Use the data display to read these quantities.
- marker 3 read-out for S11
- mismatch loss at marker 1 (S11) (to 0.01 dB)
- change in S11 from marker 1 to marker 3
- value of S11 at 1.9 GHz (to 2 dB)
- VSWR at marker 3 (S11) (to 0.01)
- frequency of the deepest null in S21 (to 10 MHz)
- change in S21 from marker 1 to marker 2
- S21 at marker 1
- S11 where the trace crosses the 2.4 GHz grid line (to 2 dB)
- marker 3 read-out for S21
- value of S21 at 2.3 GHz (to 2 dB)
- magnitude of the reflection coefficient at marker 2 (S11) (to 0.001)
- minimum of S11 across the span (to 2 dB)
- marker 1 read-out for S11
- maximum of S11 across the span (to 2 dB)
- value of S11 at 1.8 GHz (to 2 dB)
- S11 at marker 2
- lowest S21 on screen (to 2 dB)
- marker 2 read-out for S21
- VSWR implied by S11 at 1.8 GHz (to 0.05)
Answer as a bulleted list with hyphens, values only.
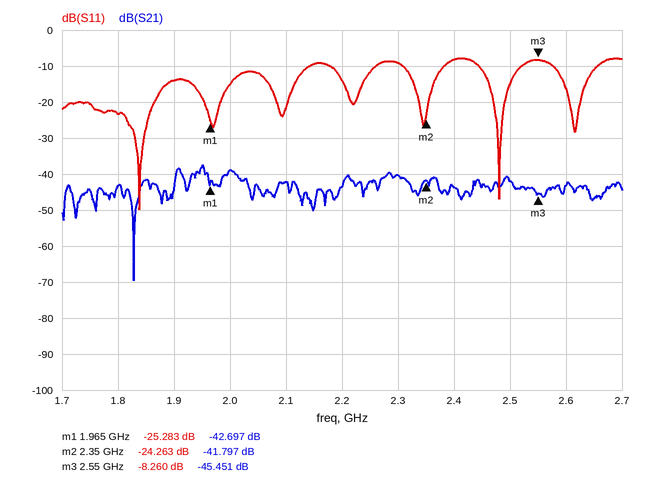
- -8.260 dB
- 0.01 dB
- 17.023 dB
- -14 dB
- 2.26
- 1.83 GHz
- 0.900 dB
- -42.697 dB
- -8 dB
- -45.451 dB
- -40 dB
- 0.061
- -50 dB
- -25.283 dB
- -8 dB
- -24 dB
- -24.263 dB
- -70 dB
- -41.797 dB
- 1.15
